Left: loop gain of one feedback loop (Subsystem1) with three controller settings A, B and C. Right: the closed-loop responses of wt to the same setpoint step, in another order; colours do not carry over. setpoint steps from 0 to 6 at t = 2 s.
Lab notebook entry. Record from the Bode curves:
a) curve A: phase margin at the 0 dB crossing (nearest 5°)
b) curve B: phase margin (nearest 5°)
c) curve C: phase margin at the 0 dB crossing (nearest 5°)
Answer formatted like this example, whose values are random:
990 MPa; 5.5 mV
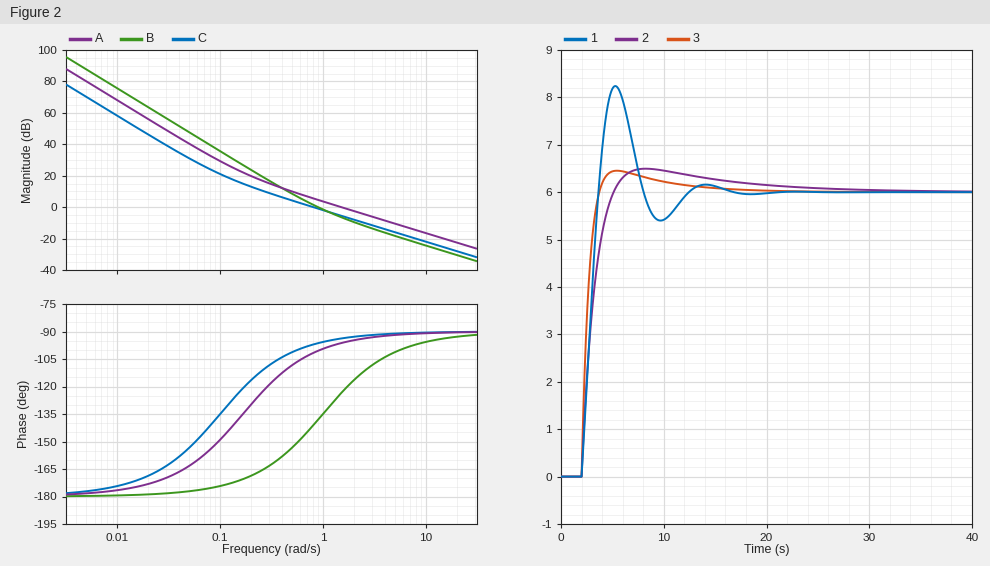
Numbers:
85°; 40°; 85°
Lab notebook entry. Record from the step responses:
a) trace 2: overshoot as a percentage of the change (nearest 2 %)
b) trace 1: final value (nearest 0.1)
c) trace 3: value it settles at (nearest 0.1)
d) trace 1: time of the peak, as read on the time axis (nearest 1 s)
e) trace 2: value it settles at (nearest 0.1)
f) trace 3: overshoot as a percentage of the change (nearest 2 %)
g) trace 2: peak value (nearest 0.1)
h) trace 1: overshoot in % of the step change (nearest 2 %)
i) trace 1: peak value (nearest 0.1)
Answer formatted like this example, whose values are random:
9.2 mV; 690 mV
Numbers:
8 %; 6.0; 6.0; 5 s; 6.0; 8 %; 6.5; 38 %; 8.2
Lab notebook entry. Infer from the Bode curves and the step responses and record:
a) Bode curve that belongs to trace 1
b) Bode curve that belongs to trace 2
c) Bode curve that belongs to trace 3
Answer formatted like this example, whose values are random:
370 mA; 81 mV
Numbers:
B; C; A
